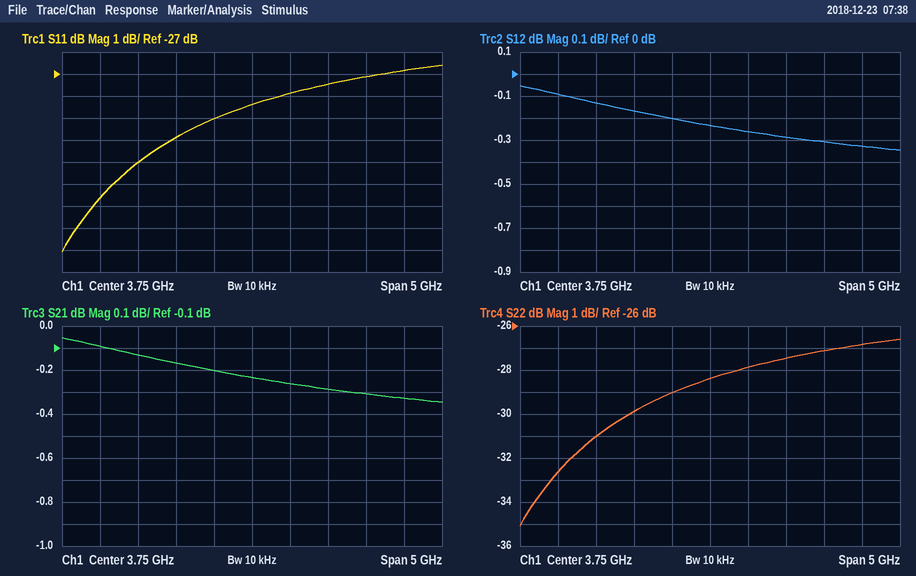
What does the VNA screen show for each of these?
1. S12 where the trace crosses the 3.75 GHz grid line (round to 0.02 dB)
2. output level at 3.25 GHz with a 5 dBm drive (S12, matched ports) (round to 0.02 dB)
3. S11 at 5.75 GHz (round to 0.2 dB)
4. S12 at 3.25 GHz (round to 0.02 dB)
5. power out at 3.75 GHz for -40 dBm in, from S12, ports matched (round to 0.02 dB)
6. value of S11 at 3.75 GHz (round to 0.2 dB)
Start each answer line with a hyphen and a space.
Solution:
- -0.24 dB
- 4.80 dBm
- -26.8 dB
- -0.20 dB
- -40.24 dBm
- -28.4 dB
